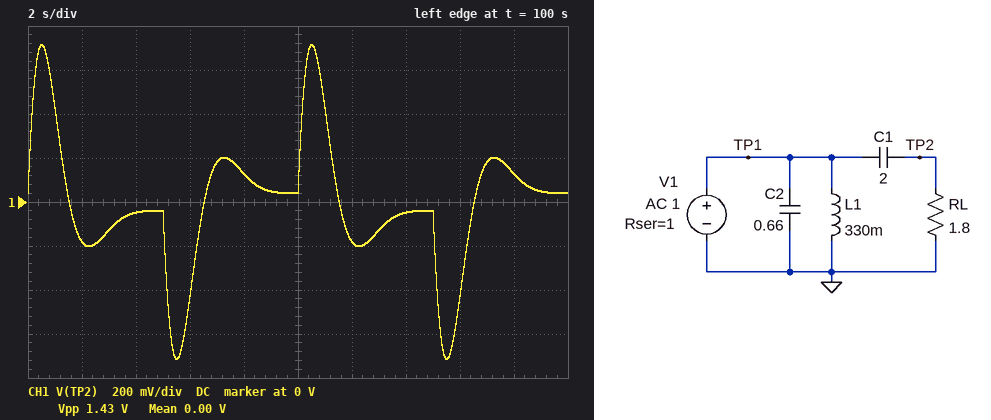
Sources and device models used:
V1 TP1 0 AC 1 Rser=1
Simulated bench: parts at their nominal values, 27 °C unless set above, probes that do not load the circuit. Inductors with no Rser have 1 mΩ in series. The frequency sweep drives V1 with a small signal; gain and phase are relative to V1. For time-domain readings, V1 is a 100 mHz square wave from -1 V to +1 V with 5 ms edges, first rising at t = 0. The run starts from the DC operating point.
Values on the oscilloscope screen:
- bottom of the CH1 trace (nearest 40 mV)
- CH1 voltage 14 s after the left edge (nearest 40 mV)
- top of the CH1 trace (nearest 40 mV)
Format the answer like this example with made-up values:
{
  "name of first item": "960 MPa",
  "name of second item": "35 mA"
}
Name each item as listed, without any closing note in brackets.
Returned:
{
  "bottom of the CH1 trace": "-720 mV",
  "CH1 voltage 14 s after the left edge": "-40 mV",
  "top of the CH1 trace": "720 mV"
}
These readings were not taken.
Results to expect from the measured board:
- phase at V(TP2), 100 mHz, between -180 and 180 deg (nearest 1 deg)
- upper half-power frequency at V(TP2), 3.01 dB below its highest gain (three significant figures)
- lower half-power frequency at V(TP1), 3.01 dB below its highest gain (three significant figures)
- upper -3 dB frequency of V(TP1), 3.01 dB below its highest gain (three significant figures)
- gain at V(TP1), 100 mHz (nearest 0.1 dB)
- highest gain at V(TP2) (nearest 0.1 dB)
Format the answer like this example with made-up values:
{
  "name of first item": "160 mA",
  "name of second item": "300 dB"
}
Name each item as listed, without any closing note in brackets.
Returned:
{
  "phase at V(TP2), 100 mHz, between -180 and 180 deg": "94 deg",
  "upper half-power frequency at V(TP2), 3.01 dB below its highest gain": "570 mHz",
  "lower half-power frequency at V(TP1), 3.01 dB below its highest gain": "194 mHz",
  "upper -3 dB frequency of V(TP1), 3.01 dB below its highest gain": "567 mHz",
  "gain at V(TP1), 100 mHz": "-13.0 dB",
  "highest gain at V(TP2)": "-3.9 dB"
}
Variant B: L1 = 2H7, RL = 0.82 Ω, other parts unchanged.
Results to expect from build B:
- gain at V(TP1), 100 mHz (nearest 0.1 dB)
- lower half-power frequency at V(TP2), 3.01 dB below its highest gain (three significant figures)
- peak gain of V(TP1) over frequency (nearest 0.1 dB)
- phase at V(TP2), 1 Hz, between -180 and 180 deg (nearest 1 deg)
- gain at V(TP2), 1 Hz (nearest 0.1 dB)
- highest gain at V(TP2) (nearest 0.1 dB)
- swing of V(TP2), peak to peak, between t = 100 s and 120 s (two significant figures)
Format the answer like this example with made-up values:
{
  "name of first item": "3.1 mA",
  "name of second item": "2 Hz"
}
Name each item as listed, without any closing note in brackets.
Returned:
{
  "gain at V(TP1), 100 mHz": "-4.5 dB",
  "lower half-power frequency at V(TP2), 3.01 dB below its highest gain": "44.7 mHz",
  "peak gain of V(TP1) over frequency": "-2.5 dB",
  "phase at V(TP2), 1 Hz, between -180 and 180 deg": "-57 deg",
  "gain at V(TP2), 1 Hz": "-13.6 dB",
  "highest gain at V(TP2)": "-7.4 dB",
  "swing of V(TP2), peak to peak, between t = 100 s and 120 s": "1.3 V"
}
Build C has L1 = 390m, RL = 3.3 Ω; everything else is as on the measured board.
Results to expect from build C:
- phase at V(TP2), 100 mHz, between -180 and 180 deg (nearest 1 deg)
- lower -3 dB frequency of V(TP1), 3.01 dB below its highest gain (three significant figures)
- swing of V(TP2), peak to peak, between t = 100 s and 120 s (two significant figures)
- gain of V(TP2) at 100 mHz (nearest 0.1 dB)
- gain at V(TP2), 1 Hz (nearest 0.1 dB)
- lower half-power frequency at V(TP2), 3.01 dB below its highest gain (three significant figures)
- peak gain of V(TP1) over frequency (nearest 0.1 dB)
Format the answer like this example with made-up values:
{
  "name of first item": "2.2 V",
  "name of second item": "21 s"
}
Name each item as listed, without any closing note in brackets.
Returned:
{
  "phase at V(TP2), 100 mHz, between -180 and 180 deg": "84 deg",
  "lower -3 dB frequency of V(TP1), 3.01 dB below its highest gain": "191 mHz",
  "swing of V(TP2), peak to peak, between t = 100 s and 120 s": "1.7 V",
  "gain of V(TP2) at 100 mHz": "-11.9 dB",
  "gain at V(TP2), 1 Hz": "-12.0 dB",
  "lower half-power frequency at V(TP2), 3.01 dB below its highest gain": "192 mHz",
  "peak gain of V(TP1) over frequency": "-2.3 dB"
}
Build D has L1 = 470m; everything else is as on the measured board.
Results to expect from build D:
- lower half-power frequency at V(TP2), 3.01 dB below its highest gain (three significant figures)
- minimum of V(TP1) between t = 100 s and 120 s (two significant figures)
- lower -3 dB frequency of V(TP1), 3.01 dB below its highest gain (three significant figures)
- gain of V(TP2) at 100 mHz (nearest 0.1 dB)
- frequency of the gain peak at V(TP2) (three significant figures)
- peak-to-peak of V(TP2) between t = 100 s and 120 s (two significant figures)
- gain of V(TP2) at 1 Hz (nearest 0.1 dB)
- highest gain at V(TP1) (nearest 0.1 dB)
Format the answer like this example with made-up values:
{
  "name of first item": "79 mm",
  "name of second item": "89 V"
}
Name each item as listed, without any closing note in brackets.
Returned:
{
  "lower half-power frequency at V(TP2), 3.01 dB below its highest gain": "150 mHz",
  "minimum of V(TP1) between t = 100 s and 120 s": "-820 mV",
  "lower -3 dB frequency of V(TP1), 3.01 dB below its highest gain": "145 mHz",
  "gain of V(TP2) at 100 mHz": "-10.7 dB",
  "frequency of the gain peak at V(TP2)": "277 mHz",
  "peak-to-peak of V(TP2) between t = 100 s and 120 s": "1.6 V",
  "gain of V(TP2) at 1 Hz": "-12.3 dB",
  "highest gain at V(TP1)": "-3.8 dB"
}
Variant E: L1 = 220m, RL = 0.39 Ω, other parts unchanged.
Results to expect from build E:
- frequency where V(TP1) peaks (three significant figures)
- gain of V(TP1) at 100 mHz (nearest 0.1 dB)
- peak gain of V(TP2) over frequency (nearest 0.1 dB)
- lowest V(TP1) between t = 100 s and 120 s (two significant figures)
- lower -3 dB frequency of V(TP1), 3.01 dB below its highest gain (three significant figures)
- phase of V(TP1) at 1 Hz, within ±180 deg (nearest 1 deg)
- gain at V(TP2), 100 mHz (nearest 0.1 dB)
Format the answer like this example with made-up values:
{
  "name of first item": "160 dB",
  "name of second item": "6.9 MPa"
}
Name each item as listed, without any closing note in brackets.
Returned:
{
  "frequency where V(TP1) peaks": "237 mHz",
  "gain of V(TP1) at 100 mHz": "-15.6 dB",
  "peak gain of V(TP2) over frequency": "-10.4 dB",
  "lowest V(TP1) between t = 100 s and 120 s": "-460 mV",
  "lower -3 dB frequency of V(TP1), 3.01 dB below its highest gain": "145 mHz",
  "phase of V(TP1) at 1 Hz, within ±180 deg": "-49 deg",
  "gain at V(TP2), 100 mHz": "-22.7 dB"
}
